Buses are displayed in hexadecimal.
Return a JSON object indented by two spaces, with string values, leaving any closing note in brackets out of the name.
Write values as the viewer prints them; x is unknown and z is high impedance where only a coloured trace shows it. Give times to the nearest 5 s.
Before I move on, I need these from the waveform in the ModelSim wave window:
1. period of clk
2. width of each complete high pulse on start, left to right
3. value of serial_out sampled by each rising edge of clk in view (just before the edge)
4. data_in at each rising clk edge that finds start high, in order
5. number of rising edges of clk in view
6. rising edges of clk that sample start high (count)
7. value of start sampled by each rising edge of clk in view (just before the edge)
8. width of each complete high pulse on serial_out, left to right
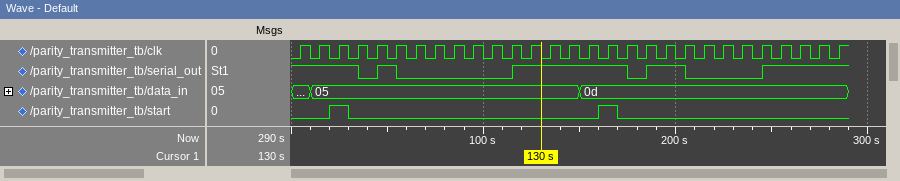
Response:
{
  "period of clk": "10 s",
  "width of each complete high pulse on start, left to right": "10 s, 10 s",
  "value of serial_out sampled by each rising edge of clk in view": "1 1 1 1 0 1 0 0 0 0 0 0 1 1 1 1 1 1 0 1 1 0 0 0 0 1 1 1 1",
  "data_in at each rising clk edge that finds start high, in order": "05, 0d",
  "number of rising edges of clk in view": "29",
  "rising edges of clk that sample start high": "2",
  "value of start sampled by each rising edge of clk in view": "0 0 1 0 0 0 0 0 0 0 0 0 0 0 0 0 1 0 0 0 0 0 0 0 0 0 0 0 0",
  "width of each complete high pulse on serial_out, left to right": "10 s, 60 s, 20 s"
}
